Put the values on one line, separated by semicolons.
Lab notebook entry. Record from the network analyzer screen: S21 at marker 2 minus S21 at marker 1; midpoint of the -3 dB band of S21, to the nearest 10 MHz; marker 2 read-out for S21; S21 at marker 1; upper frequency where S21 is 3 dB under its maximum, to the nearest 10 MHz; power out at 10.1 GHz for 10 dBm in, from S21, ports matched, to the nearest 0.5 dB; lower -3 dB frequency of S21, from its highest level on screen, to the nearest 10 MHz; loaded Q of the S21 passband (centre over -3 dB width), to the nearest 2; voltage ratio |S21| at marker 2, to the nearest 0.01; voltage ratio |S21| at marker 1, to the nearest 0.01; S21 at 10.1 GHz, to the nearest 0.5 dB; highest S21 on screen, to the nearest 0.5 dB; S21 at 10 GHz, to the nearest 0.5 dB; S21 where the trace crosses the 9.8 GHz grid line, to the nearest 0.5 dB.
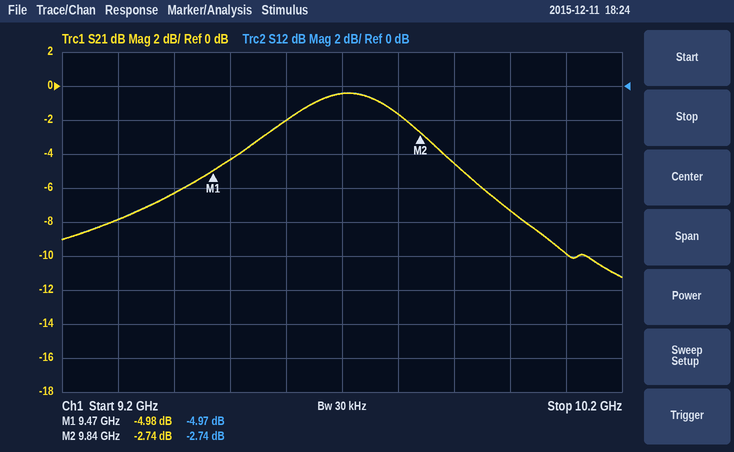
2.24 dB; 9.70 GHz; -2.74 dB; -4.98 dB; 9.86 GHz; 0.0 dBm; 9.54 GHz; 30; 0.73; 0.56; -10.0 dB; -0.5 dB; -7.5 dB; -1.5 dB
